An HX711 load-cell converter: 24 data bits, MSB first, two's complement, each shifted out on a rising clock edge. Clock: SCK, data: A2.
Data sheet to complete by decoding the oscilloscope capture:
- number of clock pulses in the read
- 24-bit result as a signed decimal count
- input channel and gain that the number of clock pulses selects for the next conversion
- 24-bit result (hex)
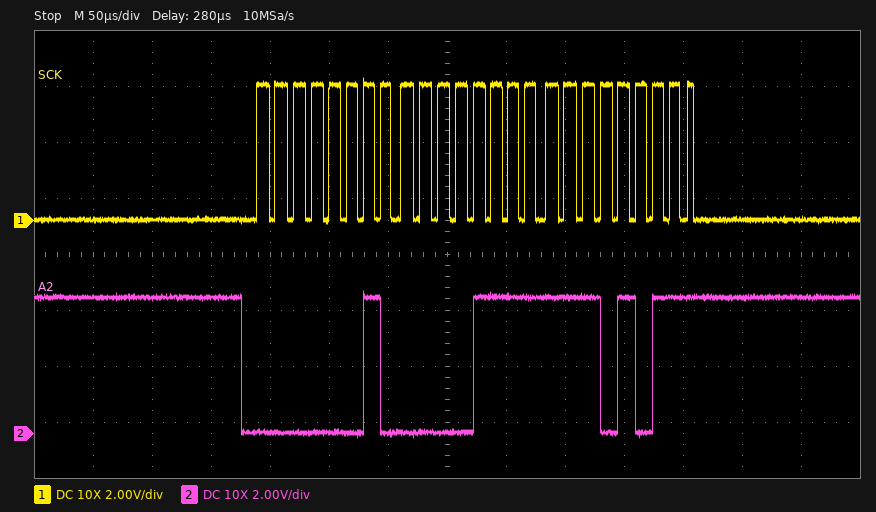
25
135147
channel A, gain 128
0x020FEB
